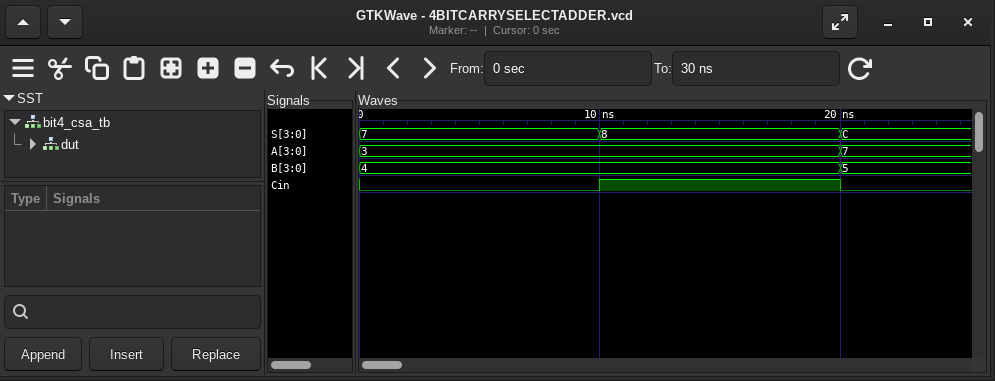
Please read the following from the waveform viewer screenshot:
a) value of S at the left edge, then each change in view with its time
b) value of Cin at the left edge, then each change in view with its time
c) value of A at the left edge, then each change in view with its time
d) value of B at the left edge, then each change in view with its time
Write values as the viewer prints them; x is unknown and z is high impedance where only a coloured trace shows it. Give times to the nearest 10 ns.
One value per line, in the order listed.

7, 8 at 10 ns, C at 20 ns
0, 1 at 10 ns, 0 at 20 ns
3, 7 at 20 ns
4, 5 at 20 ns
